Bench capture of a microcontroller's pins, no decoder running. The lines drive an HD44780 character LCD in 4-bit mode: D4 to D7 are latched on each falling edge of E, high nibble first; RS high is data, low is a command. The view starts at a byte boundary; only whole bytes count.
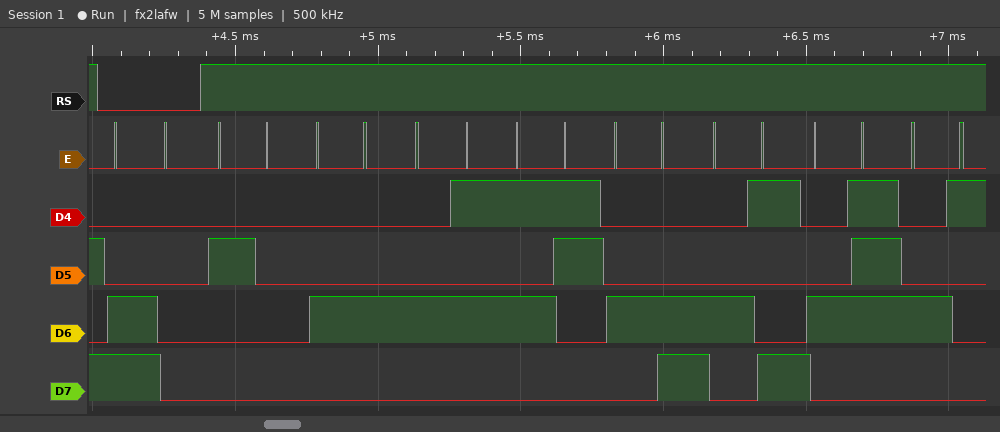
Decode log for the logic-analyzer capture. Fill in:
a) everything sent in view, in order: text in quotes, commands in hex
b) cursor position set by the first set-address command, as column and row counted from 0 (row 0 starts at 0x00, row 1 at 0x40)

0xC0 " DESLIGA"
column 0, row 1
